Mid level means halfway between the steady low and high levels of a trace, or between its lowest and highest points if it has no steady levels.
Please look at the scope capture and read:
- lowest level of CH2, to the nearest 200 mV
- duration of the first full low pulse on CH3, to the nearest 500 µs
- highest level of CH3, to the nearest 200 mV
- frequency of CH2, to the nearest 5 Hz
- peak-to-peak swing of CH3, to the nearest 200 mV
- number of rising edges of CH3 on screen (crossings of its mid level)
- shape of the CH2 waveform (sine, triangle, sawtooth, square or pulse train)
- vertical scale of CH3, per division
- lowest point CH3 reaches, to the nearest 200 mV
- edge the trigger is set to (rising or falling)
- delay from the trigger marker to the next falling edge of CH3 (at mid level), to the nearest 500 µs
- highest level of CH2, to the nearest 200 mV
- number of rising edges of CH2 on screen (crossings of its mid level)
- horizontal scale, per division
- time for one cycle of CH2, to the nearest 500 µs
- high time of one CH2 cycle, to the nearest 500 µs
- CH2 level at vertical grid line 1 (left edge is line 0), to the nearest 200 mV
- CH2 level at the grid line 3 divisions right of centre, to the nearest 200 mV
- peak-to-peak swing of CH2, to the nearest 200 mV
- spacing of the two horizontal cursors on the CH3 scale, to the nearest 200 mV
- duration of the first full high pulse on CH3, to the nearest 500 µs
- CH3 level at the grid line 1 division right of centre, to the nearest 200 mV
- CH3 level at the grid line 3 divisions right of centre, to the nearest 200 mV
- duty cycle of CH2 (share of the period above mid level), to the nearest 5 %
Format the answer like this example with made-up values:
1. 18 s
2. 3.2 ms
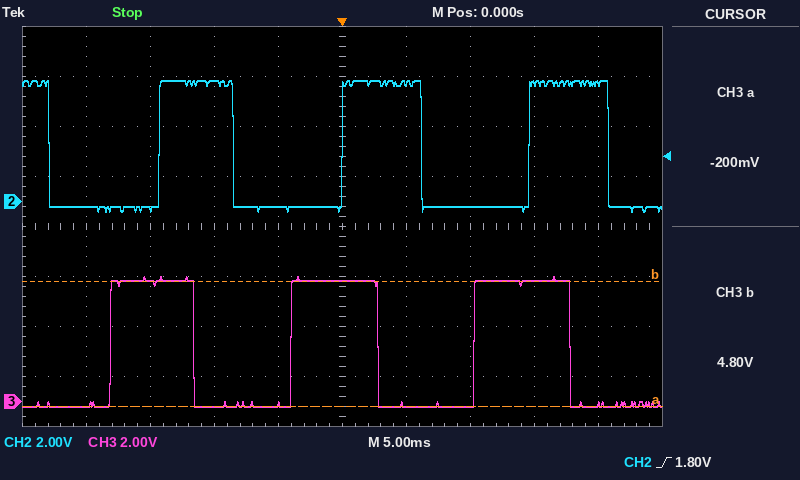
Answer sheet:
1. -400 mV
2. 7.5 ms
3. 5.0 V
4. 70 Hz
5. 5.2 V
6. 3
7. pulse train
8. 2 V
9. -200 mV
10. rising
11. 3.0 ms
12. 4.8 V
13. 3
14. 5 ms
15. 14.5 ms
16. 6.0 ms
17. -200 mV
18. 4.8 V
19. 5.2 V
20. 5.0 V
21. 6.5 ms
22. -200 mV
23. 4.8 V
24. 40 %
